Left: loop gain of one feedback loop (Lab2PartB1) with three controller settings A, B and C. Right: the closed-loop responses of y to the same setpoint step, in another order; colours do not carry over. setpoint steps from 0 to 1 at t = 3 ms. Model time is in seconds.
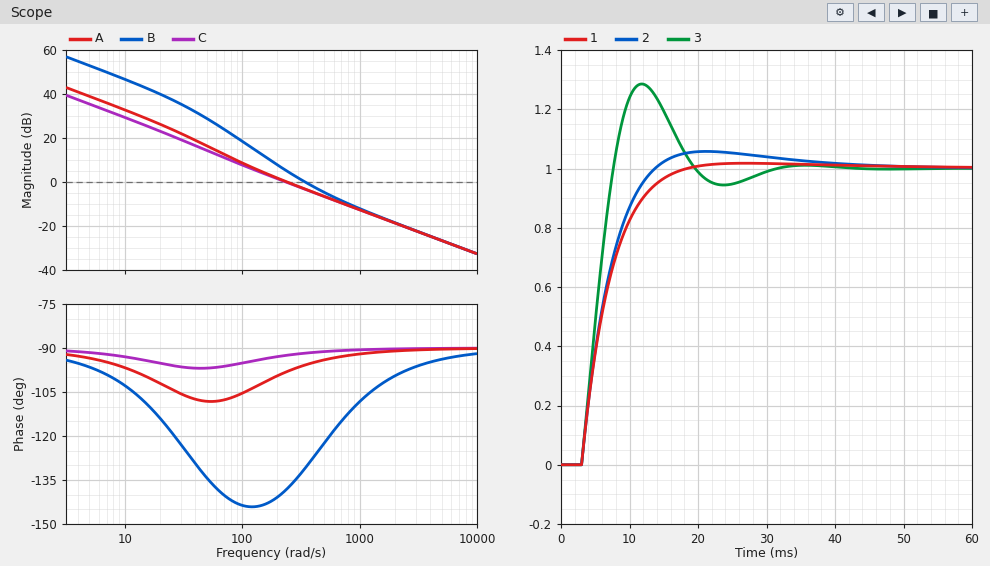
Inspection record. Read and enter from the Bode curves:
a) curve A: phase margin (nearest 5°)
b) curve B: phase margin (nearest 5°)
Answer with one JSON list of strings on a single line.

["80°", "50°"]
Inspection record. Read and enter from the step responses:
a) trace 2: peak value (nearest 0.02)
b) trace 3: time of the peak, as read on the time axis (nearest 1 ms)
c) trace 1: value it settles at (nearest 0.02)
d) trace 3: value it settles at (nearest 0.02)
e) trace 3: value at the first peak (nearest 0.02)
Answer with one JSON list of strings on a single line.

["1.06", "12 ms", "1.00", "1.00", "1.28"]
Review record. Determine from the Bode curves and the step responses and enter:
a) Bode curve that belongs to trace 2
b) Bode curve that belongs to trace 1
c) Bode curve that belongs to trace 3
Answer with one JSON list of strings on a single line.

["A", "C", "B"]
